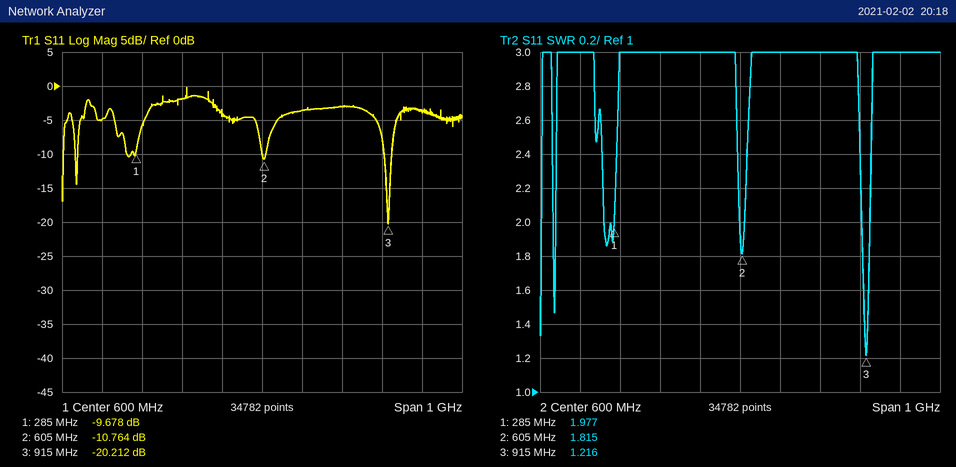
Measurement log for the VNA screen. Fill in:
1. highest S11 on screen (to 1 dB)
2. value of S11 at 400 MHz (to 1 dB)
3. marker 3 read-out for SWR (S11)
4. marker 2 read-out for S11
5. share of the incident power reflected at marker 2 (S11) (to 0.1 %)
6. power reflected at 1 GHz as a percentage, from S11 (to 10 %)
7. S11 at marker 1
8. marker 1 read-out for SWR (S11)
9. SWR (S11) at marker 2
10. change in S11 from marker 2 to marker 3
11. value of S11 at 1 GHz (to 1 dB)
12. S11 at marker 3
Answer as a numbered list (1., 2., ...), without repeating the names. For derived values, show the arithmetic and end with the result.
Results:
1. 0 dB
2. -2 dB
3. 1.216
4. -10.764 dB
5. 10^(-10.764/10) ≈ 8.4 %
6. 10^(-4/10) ≈ 40 %
7. -9.678 dB
8. 1.977
9. 1.815
10. -20.212 − (-10.764) = -9.448 dB
11. -4 dB
12. -20.212 dB
